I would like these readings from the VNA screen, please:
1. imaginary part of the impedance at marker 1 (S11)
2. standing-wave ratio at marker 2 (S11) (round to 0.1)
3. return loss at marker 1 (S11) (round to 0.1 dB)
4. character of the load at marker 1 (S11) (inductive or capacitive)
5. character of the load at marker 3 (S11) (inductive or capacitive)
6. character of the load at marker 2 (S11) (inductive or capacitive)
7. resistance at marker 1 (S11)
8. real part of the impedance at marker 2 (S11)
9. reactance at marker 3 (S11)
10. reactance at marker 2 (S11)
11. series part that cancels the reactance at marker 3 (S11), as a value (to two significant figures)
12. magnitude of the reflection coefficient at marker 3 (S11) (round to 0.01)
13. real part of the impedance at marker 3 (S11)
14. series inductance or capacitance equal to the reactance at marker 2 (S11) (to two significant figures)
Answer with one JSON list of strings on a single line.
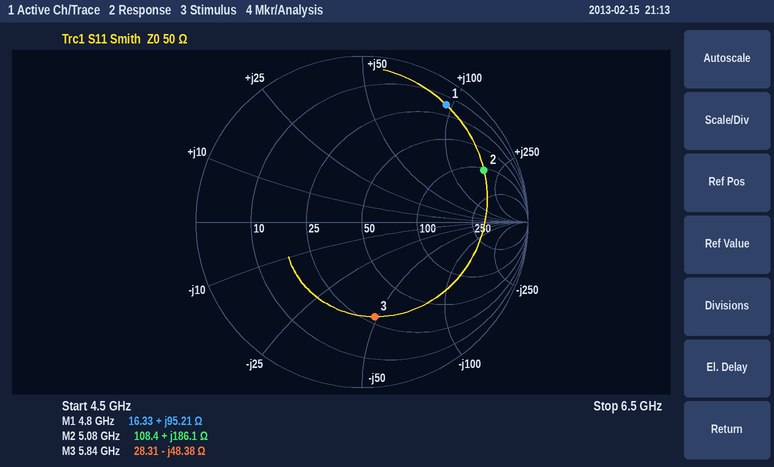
["+95.21 Ω", "8.9", "1.2 dB", "inductive", "capacitive", "inductive", "16.33 Ω", "108.4 Ω", "-48.38 Ω", "+186.1 Ω", "1.3 nH", "0.58", "28.31 Ω", "5.8 nH"]
